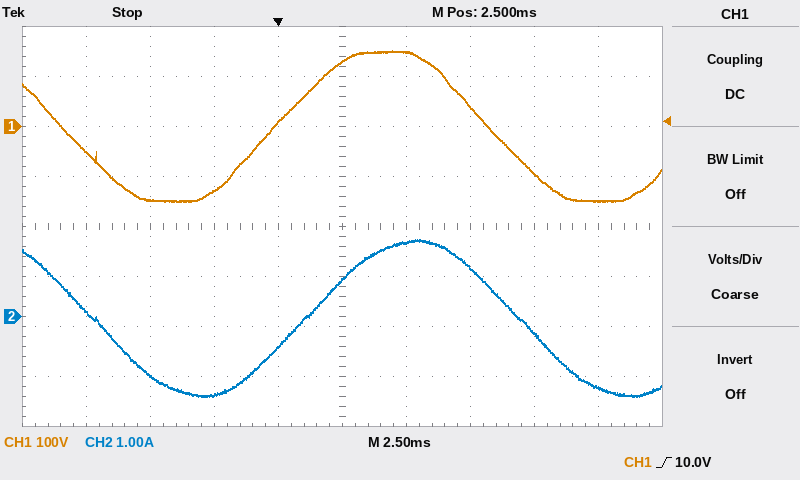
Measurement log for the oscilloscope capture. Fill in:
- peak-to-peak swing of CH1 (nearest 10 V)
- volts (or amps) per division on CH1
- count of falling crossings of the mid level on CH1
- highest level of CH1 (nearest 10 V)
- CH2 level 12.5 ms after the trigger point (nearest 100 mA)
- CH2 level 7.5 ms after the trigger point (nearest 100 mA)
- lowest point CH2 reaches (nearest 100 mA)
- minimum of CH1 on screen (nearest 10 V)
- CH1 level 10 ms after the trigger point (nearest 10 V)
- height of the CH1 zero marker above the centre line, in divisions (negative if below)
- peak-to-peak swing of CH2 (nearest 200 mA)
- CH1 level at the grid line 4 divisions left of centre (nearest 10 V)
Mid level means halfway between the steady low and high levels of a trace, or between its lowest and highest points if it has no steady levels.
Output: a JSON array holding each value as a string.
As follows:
["300 V", "100 V", "2", "150 V", "-1.4 A", "1.0 A", "-1.6 A", "-150 V", "-90 V", "+2.0 div", "3.2 A", "-50 V"]
